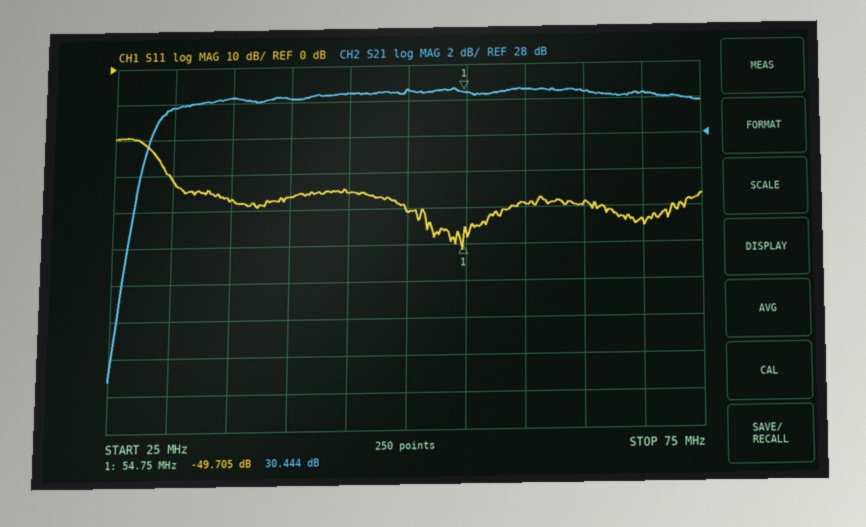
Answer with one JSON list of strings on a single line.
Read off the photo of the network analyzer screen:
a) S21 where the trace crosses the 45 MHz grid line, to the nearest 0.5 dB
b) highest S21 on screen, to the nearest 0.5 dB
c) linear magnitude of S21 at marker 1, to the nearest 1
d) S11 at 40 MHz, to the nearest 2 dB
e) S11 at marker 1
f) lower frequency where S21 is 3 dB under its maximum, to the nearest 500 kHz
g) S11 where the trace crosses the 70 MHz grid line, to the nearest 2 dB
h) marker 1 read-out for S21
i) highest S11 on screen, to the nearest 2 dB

["30.5 dB", "30.5 dB", "33", "-36 dB", "-49.705 dB", "28.0 MHz", "-44 dB", "30.444 dB", "-20 dB"]
